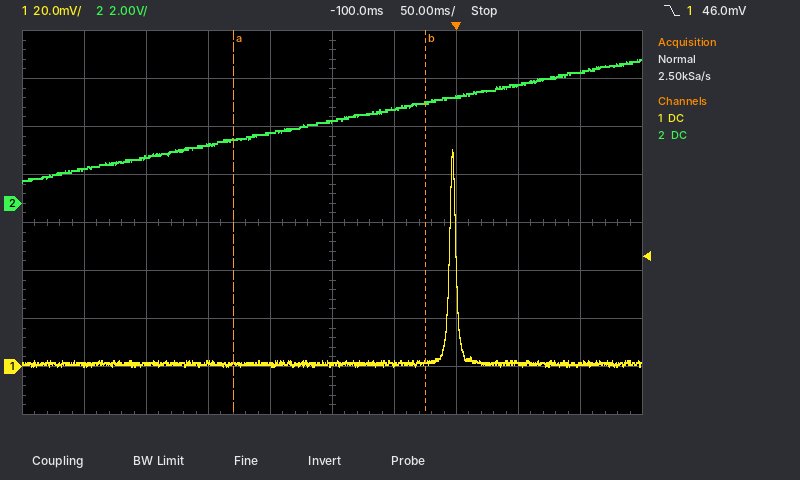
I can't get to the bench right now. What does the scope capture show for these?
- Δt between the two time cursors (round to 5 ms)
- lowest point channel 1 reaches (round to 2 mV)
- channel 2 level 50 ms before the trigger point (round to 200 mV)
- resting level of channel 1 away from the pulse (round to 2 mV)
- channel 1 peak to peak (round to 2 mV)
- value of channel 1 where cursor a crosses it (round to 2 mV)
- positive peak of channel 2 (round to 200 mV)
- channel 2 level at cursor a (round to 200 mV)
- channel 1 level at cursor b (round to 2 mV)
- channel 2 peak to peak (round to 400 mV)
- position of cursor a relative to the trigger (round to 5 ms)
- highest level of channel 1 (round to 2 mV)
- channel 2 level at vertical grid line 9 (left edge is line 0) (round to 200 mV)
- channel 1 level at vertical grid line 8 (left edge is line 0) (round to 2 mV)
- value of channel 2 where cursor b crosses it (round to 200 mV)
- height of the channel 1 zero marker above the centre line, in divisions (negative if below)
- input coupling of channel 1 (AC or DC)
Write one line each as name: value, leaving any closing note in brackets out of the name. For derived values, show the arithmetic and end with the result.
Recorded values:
Δt between the two time cursors: 155 ms
lowest point channel 1 reaches: 0 mV
channel 2 level 50 ms before the trigger point: 4.0 V
resting level of channel 1 away from the pulse: 2 mV
channel 1 peak to peak: 90 mV − (0 mV) = 90 mV
value of channel 1 where cursor a crosses it: 2 mV
positive peak of channel 2: 6.0 V
channel 2 level at cursor a: 2.6 V
channel 1 level at cursor b: 2 mV
channel 2 peak to peak: 5.2 V
position of cursor a relative to the trigger: -180 ms
highest level of channel 1: 90 mV
channel 2 level at vertical grid line 9 (left edge is line 0): 5.4 V
channel 1 level at vertical grid line 8 (left edge is line 0): 2 mV
value of channel 2 where cursor b crosses it: 4.2 V
height of the channel 1 zero marker above the centre line, in divisions: -3.0 div
input coupling of channel 1: DC
